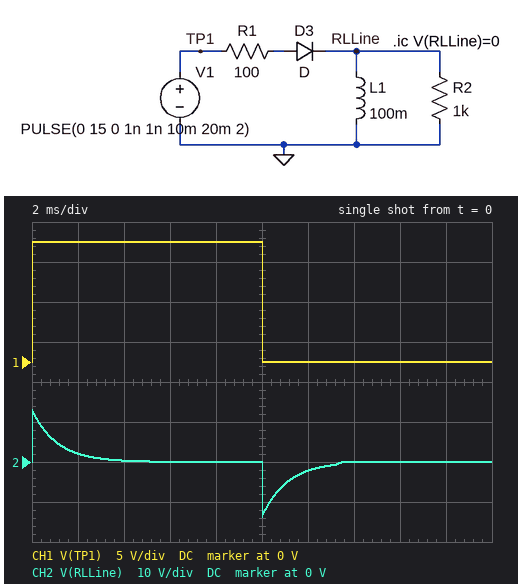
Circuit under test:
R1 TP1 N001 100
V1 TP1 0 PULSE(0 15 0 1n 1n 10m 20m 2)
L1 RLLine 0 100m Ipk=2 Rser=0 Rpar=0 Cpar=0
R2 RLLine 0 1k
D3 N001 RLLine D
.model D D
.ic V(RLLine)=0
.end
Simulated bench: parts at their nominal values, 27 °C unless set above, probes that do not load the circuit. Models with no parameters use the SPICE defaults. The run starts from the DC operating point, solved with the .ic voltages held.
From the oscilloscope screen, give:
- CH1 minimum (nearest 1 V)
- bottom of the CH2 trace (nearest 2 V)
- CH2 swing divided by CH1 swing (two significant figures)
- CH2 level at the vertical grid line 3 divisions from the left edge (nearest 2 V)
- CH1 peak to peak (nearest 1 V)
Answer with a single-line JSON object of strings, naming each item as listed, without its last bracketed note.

{"CH1 minimum": "0 V", "bottom of the CH2 trace": "-14 V", "CH2 swing divided by CH1 swing": "1.8", "CH2 level at the vertical grid line 3 divisions from the left edge": "0 V", "CH1 peak to peak": "15 V"}
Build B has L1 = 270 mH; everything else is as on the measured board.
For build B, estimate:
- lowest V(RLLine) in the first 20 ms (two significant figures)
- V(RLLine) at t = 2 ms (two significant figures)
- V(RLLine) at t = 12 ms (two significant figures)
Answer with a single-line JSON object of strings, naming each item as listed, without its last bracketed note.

{"lowest V(RLLine) in the first 20 ms": "-13 V", "V(RLLine) at t = 2 ms": "6.6 V", "V(RLLine) at t = 12 ms": "-6.7 V"}
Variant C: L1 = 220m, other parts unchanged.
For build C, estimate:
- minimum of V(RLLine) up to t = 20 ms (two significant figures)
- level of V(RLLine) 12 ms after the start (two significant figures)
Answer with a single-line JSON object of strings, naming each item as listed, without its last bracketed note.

{"minimum of V(RLLine) up to t = 20 ms": "-13 V", "level of V(RLLine) 12 ms after the start": "-5.9 V"}
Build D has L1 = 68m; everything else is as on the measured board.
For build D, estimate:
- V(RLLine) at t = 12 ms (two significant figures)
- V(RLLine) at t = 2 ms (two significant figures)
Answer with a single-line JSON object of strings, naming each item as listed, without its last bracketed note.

{"V(RLLine) at t = 12 ms": "-900 mV", "V(RLLine) at t = 2 ms": "890 mV"}
